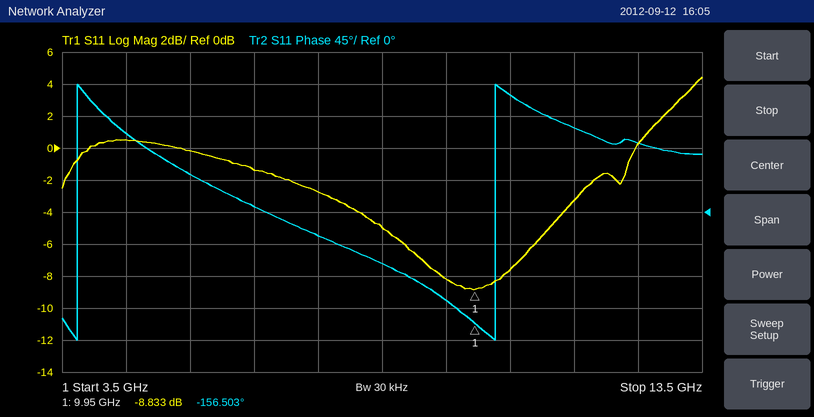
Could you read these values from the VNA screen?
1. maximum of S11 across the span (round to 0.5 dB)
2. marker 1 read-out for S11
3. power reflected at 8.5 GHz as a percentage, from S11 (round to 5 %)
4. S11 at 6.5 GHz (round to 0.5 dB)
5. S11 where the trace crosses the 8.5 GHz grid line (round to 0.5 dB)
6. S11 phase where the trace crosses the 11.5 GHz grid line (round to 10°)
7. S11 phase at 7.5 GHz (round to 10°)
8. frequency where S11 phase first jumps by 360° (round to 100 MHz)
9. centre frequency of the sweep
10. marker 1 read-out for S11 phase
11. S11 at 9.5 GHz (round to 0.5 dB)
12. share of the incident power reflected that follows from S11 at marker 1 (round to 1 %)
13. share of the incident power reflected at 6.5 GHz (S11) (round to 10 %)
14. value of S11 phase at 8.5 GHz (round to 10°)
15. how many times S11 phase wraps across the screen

4.5 dB
-8.833 dB
30 %
-1.5 dB
-5.0 dB
120°
-30°
3.7 GHz
8.5 GHz
-156.503°
-8.0 dB
13 %
70 %
-70°
2
